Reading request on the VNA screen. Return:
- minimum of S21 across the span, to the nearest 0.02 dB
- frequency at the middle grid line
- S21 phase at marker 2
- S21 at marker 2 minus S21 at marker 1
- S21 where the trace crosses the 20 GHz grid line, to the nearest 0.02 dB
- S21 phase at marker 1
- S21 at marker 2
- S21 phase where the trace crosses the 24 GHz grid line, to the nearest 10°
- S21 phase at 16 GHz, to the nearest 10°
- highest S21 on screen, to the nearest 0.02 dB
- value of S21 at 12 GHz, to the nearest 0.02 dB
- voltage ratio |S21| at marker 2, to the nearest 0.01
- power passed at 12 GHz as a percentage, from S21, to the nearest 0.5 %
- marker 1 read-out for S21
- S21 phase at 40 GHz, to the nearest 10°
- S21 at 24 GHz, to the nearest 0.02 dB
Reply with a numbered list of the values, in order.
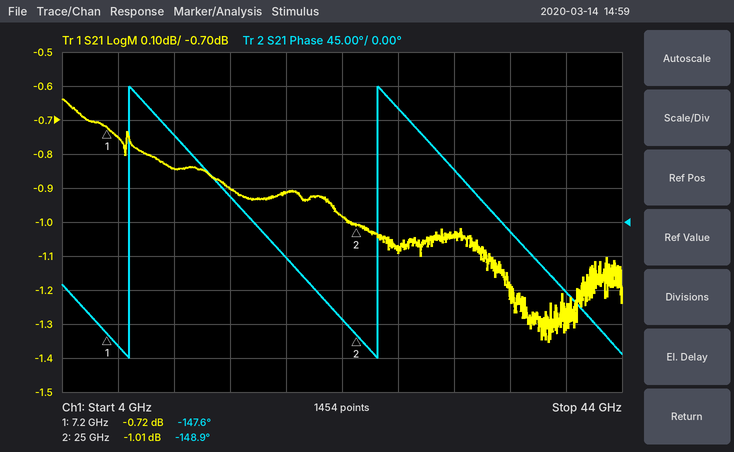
1. -1.36 dB
2. 24 GHz
3. -148.9°
4. -0.29 dB
5. -0.92 dB
6. -147.6°
7. -1.01 dB
8. -130°
9. 30°
10. -0.64 dB
11. -0.84 dB
12. 0.89
13. 82.5 %
14. -0.72 dB
15. -90°
16. -0.98 dB
